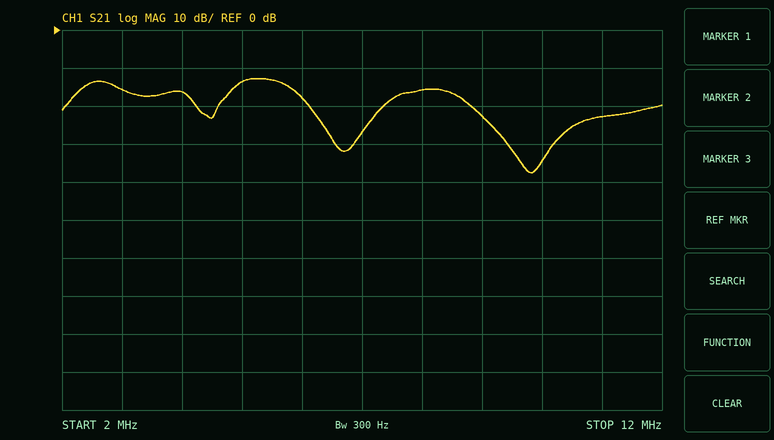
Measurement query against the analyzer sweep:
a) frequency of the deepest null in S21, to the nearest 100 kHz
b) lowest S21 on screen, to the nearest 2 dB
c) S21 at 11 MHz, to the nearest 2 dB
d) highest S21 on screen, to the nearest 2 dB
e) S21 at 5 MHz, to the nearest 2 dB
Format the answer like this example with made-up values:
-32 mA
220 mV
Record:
9.8 MHz
-38 dB
-22 dB
-12 dB
-14 dB
